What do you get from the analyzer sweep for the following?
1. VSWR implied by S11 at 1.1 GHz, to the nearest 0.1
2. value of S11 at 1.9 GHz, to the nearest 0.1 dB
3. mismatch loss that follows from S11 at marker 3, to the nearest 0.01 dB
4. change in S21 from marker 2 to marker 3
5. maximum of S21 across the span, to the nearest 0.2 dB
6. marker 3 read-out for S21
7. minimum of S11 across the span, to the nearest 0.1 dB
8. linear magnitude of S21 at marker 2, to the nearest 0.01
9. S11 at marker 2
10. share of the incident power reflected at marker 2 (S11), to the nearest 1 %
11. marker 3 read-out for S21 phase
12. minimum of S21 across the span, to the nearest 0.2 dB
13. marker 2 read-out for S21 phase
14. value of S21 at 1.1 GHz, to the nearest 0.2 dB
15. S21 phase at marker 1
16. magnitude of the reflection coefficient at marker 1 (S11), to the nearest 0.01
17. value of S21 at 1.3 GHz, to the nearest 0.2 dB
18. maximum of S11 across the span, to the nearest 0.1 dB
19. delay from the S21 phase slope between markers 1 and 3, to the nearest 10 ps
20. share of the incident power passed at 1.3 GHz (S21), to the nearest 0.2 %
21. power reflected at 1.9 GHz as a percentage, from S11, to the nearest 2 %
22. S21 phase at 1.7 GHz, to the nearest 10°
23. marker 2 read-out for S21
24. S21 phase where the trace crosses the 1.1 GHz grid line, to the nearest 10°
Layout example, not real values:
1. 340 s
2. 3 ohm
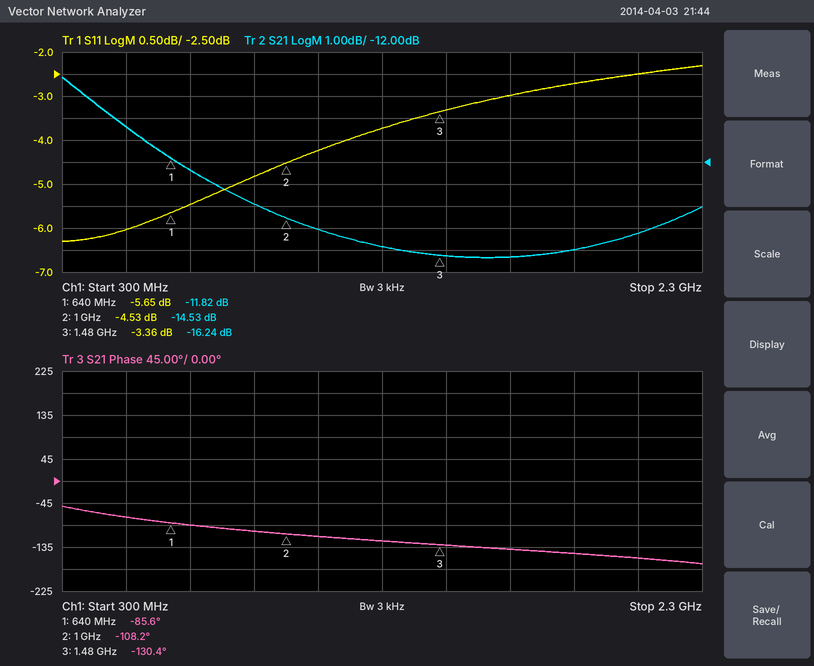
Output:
1. 4.2
2. -2.7 dB
3. 2.69 dB
4. -1.71 dB
5. -8.2 dB
6. -16.24 dB
7. -6.3 dB
8. 0.19
9. -4.53 dB
10. 35 %
11. -130.4°
12. -16.4 dB
13. -108.2°
14. -15.0 dB
15. -85.6°
16. 0.52
17. -15.8 dB
18. -2.3 dB
19. 150 ps
20. 2.6 %
21. 54 %
22. -140°
23. -14.53 dB
24. -110°
